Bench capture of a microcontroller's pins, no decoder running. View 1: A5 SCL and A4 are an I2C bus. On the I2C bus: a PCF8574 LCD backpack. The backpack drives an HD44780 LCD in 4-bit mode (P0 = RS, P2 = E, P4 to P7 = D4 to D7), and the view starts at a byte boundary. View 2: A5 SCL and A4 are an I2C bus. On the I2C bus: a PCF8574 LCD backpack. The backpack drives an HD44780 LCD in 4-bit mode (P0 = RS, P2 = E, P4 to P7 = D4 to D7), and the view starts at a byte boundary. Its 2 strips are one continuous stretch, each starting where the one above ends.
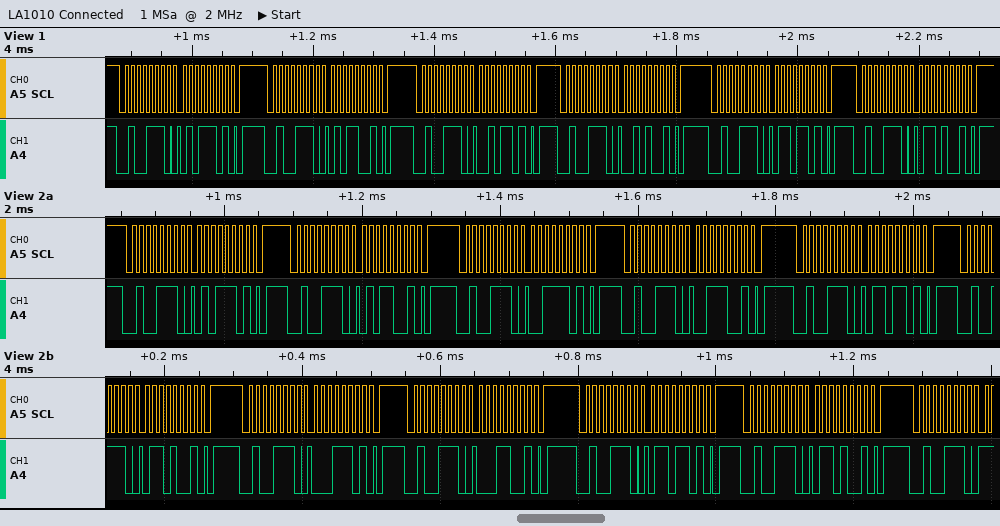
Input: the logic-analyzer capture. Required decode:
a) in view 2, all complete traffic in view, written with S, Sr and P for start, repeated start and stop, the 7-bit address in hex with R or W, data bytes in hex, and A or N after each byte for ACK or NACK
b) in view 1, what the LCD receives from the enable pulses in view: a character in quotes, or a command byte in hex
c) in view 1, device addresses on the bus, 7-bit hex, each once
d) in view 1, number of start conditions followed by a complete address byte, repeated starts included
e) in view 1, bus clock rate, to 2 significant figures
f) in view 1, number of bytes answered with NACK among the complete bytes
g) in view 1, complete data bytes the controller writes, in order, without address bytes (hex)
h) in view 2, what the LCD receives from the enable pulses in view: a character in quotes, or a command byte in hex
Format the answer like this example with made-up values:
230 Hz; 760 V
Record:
S 27W A 5D A P S 27W A 59 A P S 27W A 3D A P S 27W A 39 A P S 27W A 6D A P S 27W A 69 A P S 27W A 1D A P S 27W A 19 A P S 27W A 6D A P S 27W A 69 A P S 27W A; 'R'; 0x27; 6; 100 kHz; 0; 5D 59 2D 29 6D 69; 'S' 'a'
